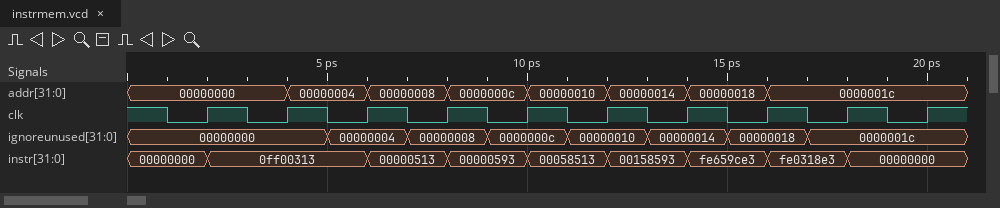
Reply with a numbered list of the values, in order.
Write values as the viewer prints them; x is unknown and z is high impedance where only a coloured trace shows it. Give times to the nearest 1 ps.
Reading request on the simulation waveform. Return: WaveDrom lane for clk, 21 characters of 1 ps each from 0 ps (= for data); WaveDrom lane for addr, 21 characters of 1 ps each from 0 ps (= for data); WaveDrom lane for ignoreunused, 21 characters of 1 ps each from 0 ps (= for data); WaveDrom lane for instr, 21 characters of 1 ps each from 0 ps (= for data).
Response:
1. {name: 'clk', wave: '101010101010101010101'}
2. {name: 'addr', wave: '=...=.=.=.=.=.=.=....', data: '00000000 00000004 00000008 0000000c 00000010 00000014 00000018 0000001c'}
3. {name: 'ignoreunused', wave: '=....=.=.=.=.=.=.=...', data: '00000000 00000004 00000008 0000000c 00000010 00000014 00000018 0000001c'}
4. {name: 'instr', wave: '=.=...=.=.=.=.=.=.=..', data: '00000000 0ff00313 00000513 00000593 00058513 00158593 fe659ce3 fe0318e3 00000000'}
